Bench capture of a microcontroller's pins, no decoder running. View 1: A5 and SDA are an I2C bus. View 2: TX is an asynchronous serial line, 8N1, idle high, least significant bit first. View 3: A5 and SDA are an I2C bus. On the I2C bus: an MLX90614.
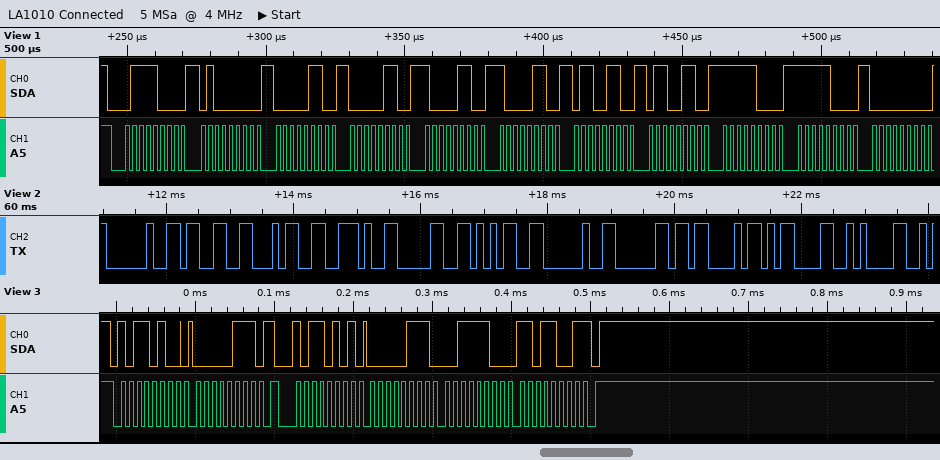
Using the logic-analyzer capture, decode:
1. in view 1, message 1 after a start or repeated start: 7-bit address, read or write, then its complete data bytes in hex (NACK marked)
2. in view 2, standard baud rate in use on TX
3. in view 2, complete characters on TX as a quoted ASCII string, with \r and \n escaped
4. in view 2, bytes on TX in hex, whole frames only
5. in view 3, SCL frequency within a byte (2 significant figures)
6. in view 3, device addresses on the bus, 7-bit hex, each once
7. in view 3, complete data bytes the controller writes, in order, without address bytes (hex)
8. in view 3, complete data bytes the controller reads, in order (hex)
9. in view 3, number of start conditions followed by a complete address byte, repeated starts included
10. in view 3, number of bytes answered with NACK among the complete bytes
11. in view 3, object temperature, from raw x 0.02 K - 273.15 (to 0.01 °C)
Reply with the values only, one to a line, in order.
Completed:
0x3C write: 40 06 06 86 86 66 66 F8 F8 00
9600 baud
" 34.05 `C\r\n"
0x20 0x33 0x34 0x2E 0x30 0x35 0x20 0x60 0x43 0x0D 0x0A
100 kHz
0x5A
07
07 3C D9
2
1
34.19 °C
